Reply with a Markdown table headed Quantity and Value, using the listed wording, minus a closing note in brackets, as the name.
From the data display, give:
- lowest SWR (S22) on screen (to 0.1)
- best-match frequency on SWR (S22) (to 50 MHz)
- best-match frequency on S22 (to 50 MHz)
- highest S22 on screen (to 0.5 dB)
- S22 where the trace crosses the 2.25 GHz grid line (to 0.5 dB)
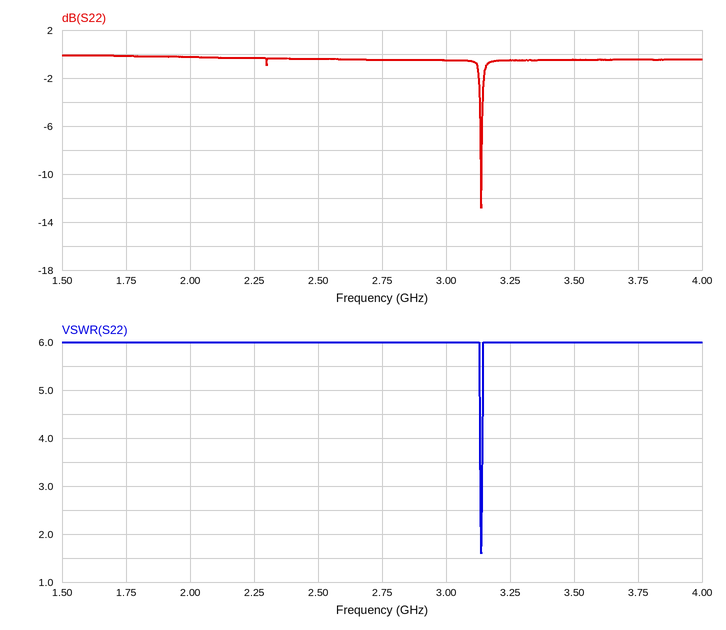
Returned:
| Quantity | Value |
|---|---|
| lowest SWR (S22) on screen | 1.6 |
| best-match frequency on SWR (S22) | 3.15 GHz |
| best-match frequency on S22 | 3.15 GHz |
| highest S22 on screen | 0.0 dB |
| S22 where the trace crosses the 2.25 GHz grid line | -0.5 dB |
